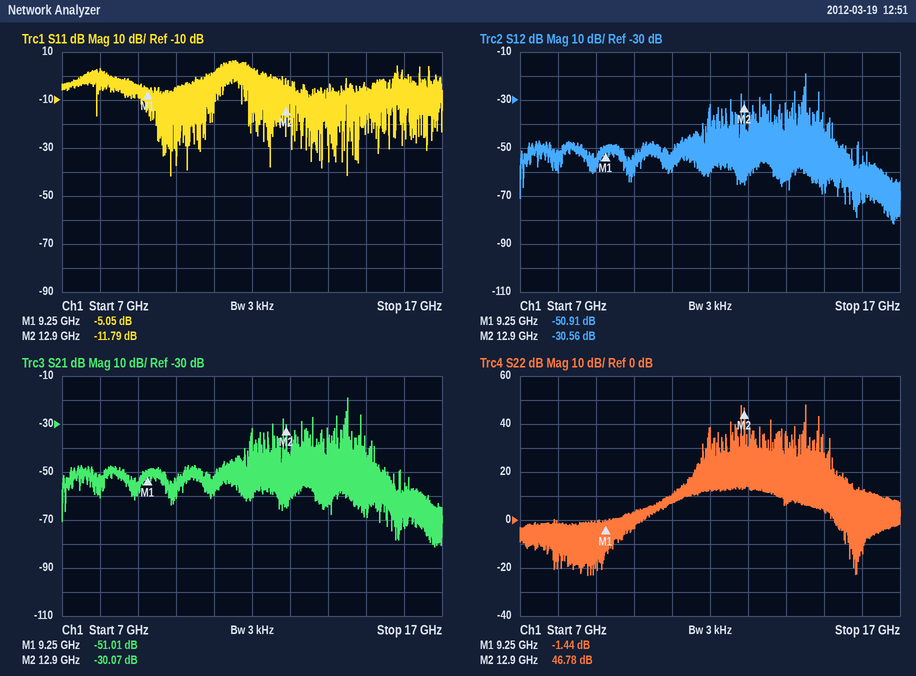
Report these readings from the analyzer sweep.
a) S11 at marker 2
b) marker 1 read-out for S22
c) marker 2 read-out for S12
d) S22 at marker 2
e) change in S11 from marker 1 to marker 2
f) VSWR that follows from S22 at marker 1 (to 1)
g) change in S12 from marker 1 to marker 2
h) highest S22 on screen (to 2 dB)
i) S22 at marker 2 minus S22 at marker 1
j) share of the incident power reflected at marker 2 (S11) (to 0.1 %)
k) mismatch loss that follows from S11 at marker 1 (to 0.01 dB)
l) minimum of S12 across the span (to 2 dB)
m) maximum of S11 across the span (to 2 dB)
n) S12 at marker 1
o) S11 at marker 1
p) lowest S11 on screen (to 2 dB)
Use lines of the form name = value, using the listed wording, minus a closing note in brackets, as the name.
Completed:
S11 at marker 2 = -11.79 dB
marker 1 read-out for S22 = -1.44 dB
marker 2 read-out for S12 = -30.56 dB
S22 at marker 2 = 46.78 dB
change in S11 from marker 1 to marker 2 = -6.74 dB
VSWR that follows from S22 at marker 1 = 12
change in S12 from marker 1 to marker 2 = 20.35 dB
highest S22 on screen = 48 dB
S22 at marker 2 minus S22 at marker 1 = 48.22 dB
share of the incident power reflected at marker 2 (S11) = 6.6 %
mismatch loss that follows from S11 at marker 1 = 1.63 dB
minimum of S12 across the span = -82 dB
maximum of S11 across the span = 6 dB
S12 at marker 1 = -50.91 dB
S11 at marker 1 = -5.05 dB
lowest S11 on screen = -42 dB
